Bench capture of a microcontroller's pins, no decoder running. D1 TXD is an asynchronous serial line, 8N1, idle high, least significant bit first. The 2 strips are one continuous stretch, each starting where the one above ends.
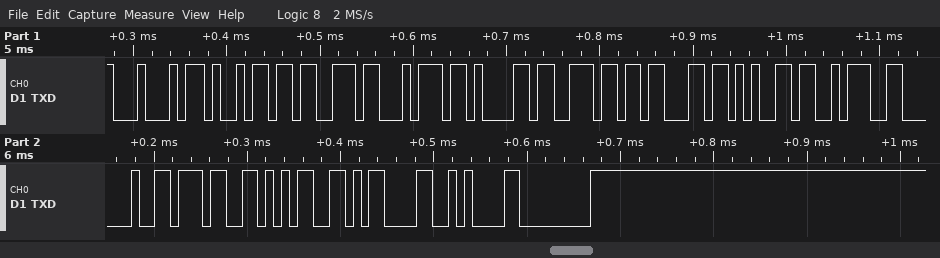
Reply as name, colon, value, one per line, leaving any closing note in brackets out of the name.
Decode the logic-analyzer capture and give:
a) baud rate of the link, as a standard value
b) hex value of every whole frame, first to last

baud rate of the link, as a standard value: 115200 baud
hex value of every whole frame, first to last: 44 69 73 74 61 6E 63 65 3A 20 37 35 0D 0A 00
